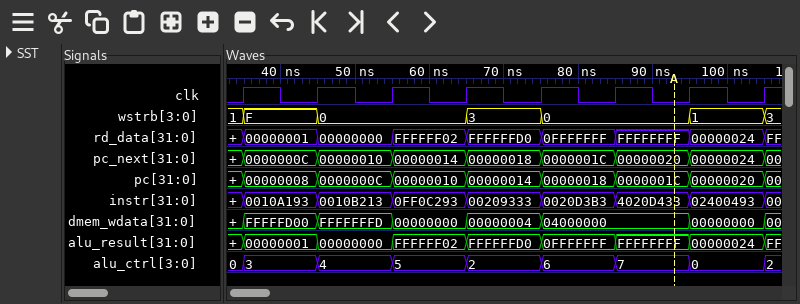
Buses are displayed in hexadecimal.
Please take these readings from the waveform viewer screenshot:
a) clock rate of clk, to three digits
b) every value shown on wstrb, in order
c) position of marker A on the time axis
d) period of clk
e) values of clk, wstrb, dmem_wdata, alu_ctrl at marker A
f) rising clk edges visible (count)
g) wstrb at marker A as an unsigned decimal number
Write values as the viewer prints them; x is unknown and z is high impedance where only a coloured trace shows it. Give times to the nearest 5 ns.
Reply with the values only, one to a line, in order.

100 MHz
1, F, 0, 3, 0, 1, 3
95 ns
10 ns
clk=0, wstrb=0, dmem_wdata=04000000, alu_ctrl=7
8
0
